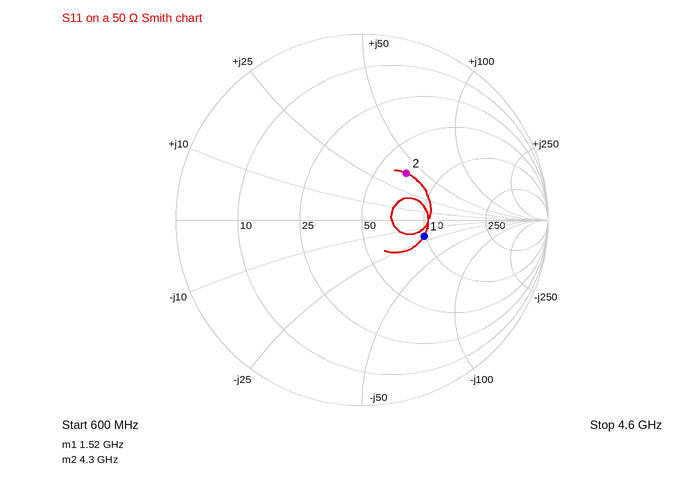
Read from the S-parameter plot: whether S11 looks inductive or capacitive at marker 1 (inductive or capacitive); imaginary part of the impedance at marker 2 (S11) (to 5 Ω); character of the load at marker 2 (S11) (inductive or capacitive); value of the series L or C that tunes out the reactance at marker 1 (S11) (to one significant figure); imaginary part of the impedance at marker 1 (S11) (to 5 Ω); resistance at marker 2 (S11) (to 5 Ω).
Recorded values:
capacitive
+40 Ω
inductive
2 nH
-20 Ω
70 Ω
